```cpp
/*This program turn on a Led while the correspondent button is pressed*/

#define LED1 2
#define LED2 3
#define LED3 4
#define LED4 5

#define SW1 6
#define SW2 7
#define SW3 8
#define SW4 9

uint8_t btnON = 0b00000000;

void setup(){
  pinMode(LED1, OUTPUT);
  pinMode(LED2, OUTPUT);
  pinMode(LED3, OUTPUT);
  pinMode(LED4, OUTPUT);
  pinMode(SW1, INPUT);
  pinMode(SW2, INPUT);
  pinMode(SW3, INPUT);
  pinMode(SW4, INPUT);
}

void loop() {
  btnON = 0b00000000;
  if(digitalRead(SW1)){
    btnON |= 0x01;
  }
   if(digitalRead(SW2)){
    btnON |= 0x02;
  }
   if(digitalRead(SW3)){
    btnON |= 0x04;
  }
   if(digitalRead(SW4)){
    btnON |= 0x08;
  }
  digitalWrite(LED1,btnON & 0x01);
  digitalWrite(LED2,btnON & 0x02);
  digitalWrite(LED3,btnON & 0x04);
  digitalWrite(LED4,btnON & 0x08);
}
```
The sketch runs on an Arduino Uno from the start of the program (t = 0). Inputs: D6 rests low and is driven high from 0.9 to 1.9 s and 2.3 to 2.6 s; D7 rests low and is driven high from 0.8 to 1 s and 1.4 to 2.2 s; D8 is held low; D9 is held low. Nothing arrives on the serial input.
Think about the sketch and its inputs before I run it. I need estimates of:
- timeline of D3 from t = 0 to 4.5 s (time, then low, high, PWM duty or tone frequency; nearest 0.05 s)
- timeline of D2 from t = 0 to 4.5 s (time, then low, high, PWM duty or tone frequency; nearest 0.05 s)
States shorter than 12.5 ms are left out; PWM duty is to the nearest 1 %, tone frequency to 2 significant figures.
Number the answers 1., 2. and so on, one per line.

1. 0 s low; 0.8 s high; 1 s low; 1.4 s high; 2.2 s low
2. 0 s low; 0.9 s high; 1.9 s low; 2.3 s high; 2.6 s low
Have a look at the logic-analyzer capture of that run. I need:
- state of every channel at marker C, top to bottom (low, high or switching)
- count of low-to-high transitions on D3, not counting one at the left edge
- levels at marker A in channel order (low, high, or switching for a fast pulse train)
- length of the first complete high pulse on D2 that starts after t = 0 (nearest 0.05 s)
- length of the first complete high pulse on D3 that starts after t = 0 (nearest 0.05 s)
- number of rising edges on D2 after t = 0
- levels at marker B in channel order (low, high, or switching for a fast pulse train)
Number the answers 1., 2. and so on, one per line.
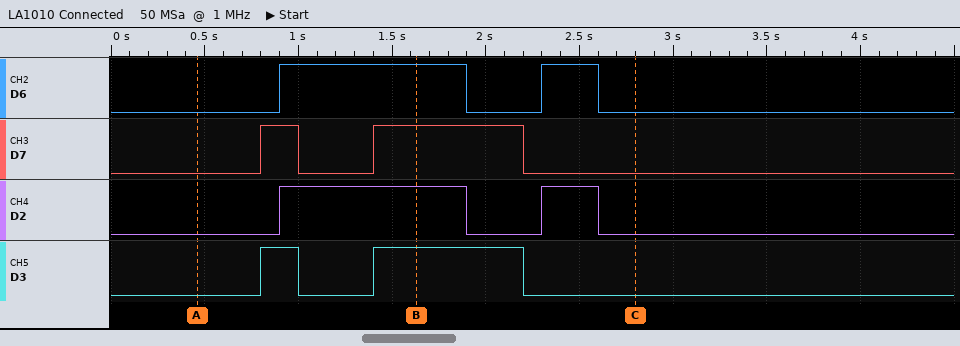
1. D6 low, D7 low, D2 low, D3 low
2. 2
3. D6 low, D7 low, D2 low, D3 low
4. 1.00 s
5. 0.20 s
6. 2
7. D6 high, D7 high, D2 high, D3 high
